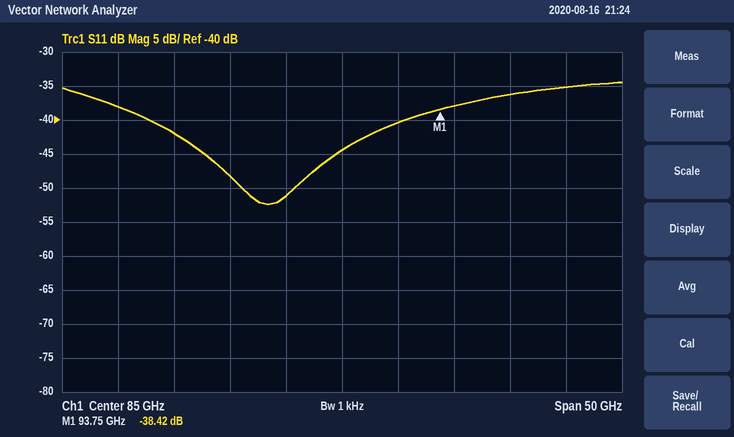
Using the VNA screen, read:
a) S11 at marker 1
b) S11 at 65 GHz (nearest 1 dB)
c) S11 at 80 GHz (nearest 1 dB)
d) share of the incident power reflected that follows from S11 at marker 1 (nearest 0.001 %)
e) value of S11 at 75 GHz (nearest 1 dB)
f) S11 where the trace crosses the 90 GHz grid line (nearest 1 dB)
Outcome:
-38.42 dB
-38 dB
-51 dB
0.014 %
-48 dB
-40 dB
